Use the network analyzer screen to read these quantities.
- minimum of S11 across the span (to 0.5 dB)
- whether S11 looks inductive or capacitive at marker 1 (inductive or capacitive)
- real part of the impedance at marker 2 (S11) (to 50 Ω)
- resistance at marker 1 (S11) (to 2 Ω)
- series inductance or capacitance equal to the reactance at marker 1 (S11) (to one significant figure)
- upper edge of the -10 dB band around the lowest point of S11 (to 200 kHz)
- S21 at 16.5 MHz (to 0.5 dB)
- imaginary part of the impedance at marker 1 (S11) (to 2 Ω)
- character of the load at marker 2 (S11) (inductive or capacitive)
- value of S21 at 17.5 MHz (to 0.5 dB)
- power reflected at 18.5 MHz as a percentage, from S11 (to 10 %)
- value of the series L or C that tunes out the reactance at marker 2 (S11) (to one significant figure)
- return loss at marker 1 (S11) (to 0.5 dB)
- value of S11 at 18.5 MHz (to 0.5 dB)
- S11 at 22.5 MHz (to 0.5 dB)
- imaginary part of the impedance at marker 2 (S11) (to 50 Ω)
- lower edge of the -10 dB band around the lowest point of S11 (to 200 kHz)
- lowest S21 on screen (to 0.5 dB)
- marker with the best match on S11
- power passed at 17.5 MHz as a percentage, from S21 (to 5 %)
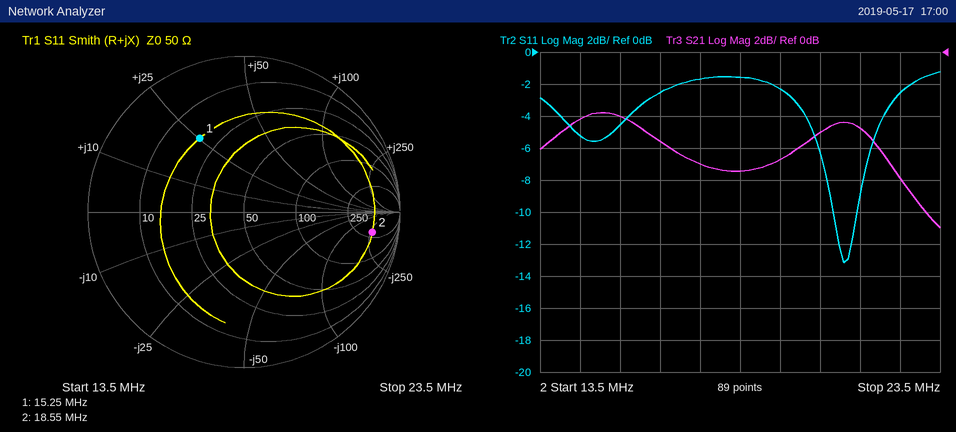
-13.0 dB
inductive
300 Ω
18 Ω
300 nH
21.4 MHz
-5.5 dB
+26 Ω
capacitive
-7.0 dB
70 %
2 µH
5.0 dB
-1.5 dB
-2.5 dB
-250 Ω
20.8 MHz
-11.0 dB
marker 1
20 %
